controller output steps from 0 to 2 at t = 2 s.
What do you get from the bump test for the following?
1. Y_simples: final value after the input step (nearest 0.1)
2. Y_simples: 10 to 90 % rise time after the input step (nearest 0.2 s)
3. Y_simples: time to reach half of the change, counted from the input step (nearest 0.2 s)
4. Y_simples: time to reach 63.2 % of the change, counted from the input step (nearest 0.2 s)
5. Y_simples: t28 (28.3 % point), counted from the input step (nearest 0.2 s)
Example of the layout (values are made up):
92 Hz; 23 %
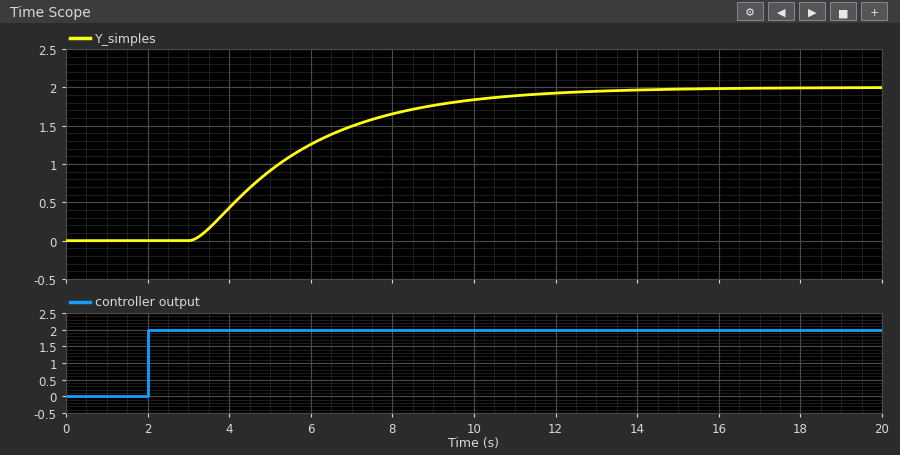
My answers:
2.0; 5.8 s; 3.2 s; 4.0 s; 2.2 s
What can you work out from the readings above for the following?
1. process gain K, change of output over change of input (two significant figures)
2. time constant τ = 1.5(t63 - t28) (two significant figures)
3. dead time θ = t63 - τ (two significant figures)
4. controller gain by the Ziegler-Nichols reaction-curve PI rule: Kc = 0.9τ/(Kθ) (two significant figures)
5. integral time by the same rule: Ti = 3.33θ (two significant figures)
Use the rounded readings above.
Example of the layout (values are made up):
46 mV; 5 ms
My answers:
1.0; 2.7 s; 1.3 s; 1.9; 4.3 s
